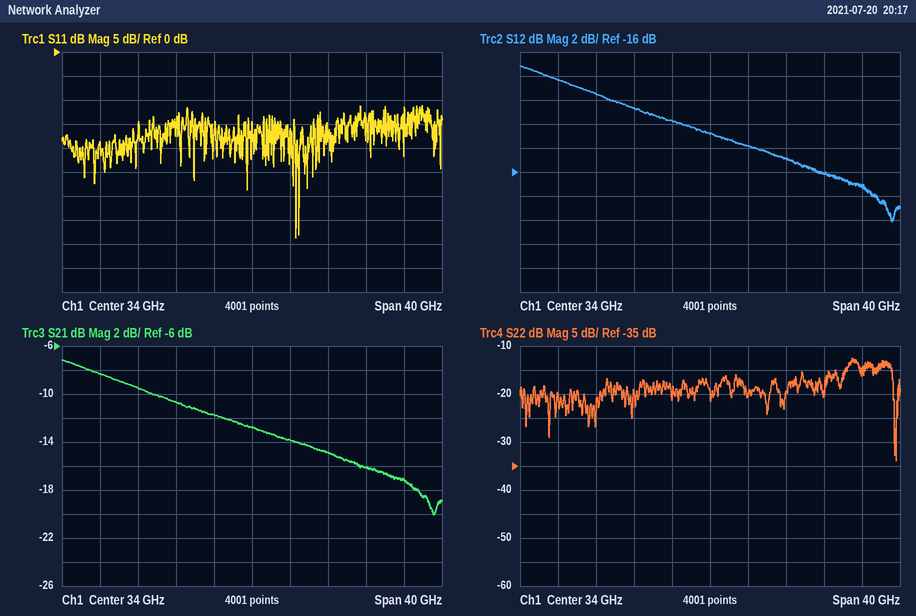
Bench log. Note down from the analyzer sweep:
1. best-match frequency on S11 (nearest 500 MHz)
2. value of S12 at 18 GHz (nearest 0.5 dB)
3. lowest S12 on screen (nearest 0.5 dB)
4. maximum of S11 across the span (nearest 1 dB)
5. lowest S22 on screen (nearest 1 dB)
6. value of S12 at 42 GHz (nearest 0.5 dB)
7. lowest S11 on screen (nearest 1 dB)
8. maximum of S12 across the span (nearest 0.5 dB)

38.5 GHz
-8.5 dB
-20.0 dB
-11 dB
-34 dB
-15.0 dB
-39 dB
-7.0 dB
